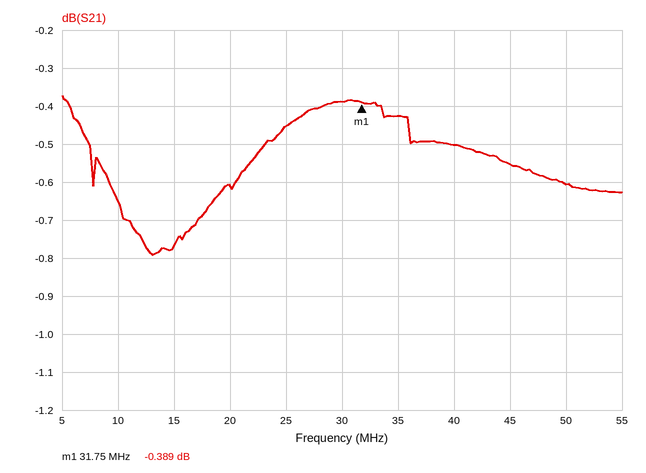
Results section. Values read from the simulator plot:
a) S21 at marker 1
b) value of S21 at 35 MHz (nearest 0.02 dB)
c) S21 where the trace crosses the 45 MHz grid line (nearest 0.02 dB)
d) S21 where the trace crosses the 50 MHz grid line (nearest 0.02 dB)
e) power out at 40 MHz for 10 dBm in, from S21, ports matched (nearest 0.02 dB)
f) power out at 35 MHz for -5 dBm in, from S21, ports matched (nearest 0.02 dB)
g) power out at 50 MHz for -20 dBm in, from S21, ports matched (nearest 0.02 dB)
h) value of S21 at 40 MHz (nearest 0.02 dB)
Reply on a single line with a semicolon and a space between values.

-0.389 dB; -0.42 dB; -0.56 dB; -0.60 dB; 9.50 dBm; -5.42 dBm; -20.60 dBm; -0.50 dB
